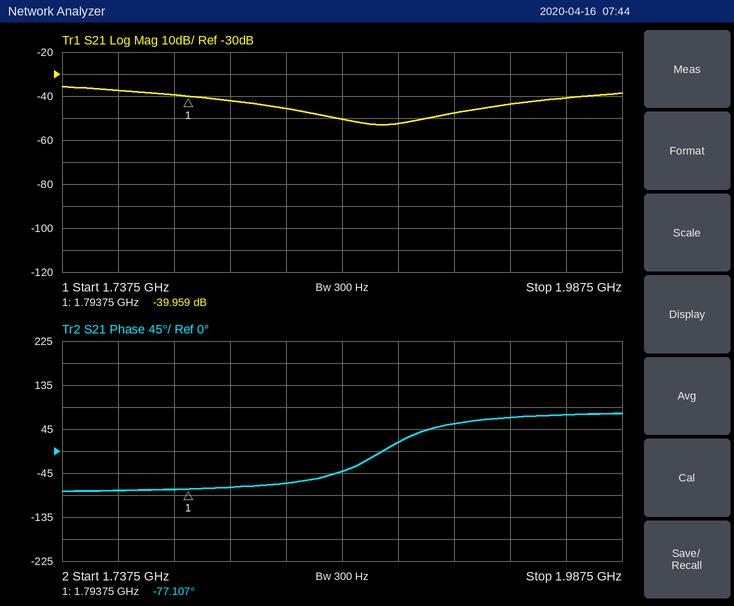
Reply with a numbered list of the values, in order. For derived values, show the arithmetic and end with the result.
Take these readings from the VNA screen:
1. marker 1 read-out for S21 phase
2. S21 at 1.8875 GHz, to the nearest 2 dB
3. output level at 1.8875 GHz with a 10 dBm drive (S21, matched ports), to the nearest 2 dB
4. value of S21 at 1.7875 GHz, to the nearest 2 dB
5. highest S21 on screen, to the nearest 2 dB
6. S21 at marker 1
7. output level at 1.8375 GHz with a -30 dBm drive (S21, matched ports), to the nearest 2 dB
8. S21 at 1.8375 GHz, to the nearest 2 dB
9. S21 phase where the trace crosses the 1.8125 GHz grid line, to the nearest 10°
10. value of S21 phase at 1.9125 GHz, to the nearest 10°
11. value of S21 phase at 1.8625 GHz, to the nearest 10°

1. -77.107°
2. -52 dB
3. 10 dBm + (-52 dB) = -42 dBm
4. -40 dB
5. -36 dB
6. -39.959 dB
7. -30 dBm + (-46 dB) = -76 dBm
8. -46 dB
9. -70°
10. 60°
11. -40°
